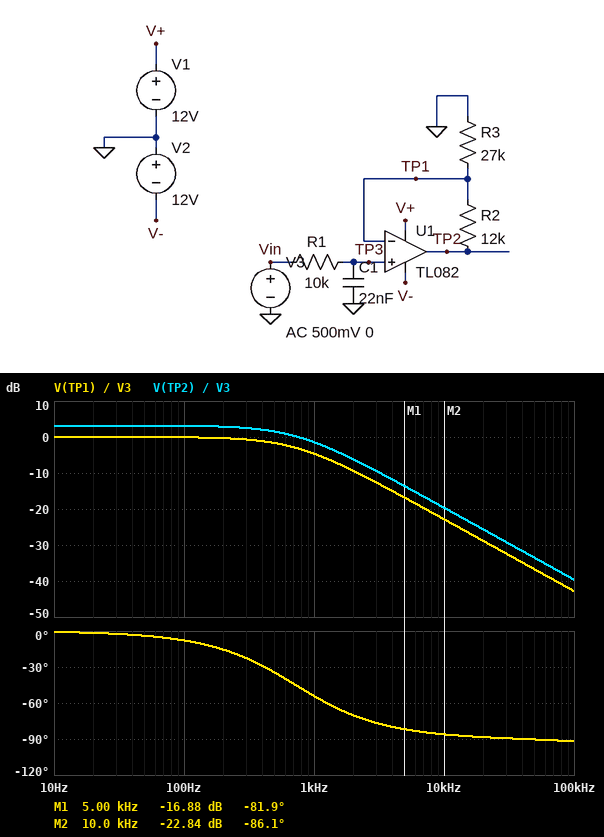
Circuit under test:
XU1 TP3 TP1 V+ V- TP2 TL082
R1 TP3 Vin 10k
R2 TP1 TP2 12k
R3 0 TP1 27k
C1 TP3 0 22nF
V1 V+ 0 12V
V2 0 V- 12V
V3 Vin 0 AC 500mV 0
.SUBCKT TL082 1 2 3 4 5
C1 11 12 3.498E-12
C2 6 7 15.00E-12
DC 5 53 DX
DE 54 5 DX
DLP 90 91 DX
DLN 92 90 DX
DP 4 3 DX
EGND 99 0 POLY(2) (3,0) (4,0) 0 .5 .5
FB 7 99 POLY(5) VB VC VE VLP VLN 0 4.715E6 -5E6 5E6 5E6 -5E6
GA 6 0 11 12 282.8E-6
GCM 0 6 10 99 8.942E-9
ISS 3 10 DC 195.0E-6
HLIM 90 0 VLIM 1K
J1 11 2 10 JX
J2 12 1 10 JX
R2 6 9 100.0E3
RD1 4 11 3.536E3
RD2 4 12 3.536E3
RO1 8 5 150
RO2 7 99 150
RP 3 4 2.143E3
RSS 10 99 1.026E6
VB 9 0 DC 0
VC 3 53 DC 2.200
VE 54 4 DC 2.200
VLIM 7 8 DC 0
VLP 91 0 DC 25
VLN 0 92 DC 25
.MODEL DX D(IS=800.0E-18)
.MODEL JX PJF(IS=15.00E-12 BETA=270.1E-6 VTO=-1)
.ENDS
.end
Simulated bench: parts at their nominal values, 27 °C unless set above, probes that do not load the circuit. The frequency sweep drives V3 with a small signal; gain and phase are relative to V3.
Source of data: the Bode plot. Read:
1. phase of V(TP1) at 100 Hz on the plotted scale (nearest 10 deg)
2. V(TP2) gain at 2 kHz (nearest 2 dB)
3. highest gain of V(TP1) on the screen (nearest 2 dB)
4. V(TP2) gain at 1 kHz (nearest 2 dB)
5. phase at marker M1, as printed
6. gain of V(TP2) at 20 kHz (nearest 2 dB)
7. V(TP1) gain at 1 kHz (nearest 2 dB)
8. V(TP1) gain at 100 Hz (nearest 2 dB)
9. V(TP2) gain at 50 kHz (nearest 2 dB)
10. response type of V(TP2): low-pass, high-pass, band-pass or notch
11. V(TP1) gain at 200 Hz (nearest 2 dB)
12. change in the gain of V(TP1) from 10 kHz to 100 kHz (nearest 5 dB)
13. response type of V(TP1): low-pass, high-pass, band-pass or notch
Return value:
-10 deg
-6 dB
0 dB
-2 dB
-81.9 deg
-26 dB
-4 dB
0 dB
-34 dB
low-pass
0 dB
-20 dB
low-pass
